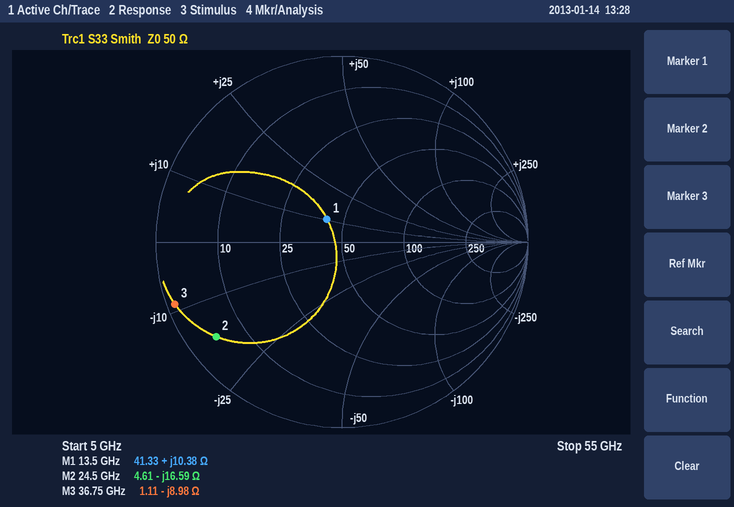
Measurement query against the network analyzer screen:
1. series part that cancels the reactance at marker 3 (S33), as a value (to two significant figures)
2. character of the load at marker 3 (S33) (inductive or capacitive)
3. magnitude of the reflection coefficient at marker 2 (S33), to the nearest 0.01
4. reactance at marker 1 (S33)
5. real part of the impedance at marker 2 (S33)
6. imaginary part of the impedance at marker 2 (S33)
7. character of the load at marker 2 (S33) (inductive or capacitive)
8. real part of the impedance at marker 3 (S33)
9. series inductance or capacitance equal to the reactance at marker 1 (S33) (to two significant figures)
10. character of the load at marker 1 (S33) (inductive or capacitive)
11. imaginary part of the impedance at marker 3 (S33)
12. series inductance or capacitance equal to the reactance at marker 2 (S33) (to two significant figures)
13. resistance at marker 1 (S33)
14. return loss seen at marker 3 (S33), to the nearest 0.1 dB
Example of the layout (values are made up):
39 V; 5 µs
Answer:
39 pH; capacitive; 0.85; +10.38 Ω; 4.61 Ω; -16.59 Ω; capacitive; 1.11 Ω; 120 pH; inductive; -8.98 Ω; 390 fF; 41.33 Ω; 0.4 dB
